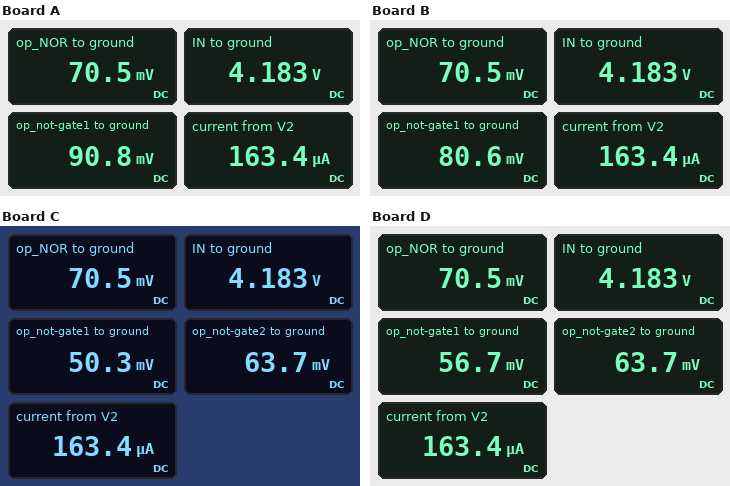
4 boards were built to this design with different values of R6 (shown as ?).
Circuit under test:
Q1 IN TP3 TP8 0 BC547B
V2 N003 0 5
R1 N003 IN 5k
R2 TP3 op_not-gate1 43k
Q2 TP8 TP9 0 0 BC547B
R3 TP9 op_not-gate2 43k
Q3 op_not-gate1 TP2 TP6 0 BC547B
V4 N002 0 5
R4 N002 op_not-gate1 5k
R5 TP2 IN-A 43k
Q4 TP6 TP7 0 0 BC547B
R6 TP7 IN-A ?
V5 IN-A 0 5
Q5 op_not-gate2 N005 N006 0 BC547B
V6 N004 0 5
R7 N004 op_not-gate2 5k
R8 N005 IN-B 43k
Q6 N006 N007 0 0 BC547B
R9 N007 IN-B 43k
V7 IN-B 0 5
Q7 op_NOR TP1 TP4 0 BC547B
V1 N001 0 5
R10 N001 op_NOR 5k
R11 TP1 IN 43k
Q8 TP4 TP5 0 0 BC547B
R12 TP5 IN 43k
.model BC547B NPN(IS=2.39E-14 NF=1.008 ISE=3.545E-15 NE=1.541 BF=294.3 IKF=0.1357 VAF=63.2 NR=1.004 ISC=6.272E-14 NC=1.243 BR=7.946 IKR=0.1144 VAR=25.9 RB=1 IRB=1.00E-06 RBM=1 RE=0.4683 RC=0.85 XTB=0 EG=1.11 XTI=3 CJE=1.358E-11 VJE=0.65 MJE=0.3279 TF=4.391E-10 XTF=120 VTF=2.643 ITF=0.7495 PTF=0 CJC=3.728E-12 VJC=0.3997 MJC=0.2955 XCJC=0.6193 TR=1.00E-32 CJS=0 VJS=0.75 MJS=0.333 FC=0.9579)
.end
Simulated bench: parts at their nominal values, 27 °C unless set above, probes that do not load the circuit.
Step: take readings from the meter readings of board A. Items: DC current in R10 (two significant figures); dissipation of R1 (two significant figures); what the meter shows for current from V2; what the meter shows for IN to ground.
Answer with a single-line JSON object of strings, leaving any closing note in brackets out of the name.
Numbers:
{"DC current in R10": "990 µA", "dissipation of R1": "130 µW", "what the meter shows for current from V2": "163.4 µA", "what the meter shows for IN to ground": "4.183 V"}
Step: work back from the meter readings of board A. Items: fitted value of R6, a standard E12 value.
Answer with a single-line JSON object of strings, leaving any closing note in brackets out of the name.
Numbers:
{"fitted value of R6, a standard E12 value": "150 kΩ"}
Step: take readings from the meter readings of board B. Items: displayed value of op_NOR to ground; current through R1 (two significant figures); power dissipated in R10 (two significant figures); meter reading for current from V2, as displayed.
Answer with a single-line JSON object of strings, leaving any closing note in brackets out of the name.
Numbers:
{"displayed value of op_NOR to ground": "70.5 mV", "current through R1": "160 µA", "power dissipated in R10": "4.9 mW", "meter reading for current from V2, as displayed": "163.4 µA"}
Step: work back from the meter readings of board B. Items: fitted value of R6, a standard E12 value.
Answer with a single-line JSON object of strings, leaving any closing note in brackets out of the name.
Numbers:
{"fitted value of R6, a standard E12 value": "100 kΩ"}
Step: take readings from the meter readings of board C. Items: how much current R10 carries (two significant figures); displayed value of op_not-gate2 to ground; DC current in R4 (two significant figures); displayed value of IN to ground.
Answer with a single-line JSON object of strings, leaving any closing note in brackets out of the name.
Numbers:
{"how much current R10 carries": "990 µA", "displayed value of op_not-gate2 to ground": "63.7 mV", "DC current in R4": "990 µA", "displayed value of IN to ground": "4.183 V"}
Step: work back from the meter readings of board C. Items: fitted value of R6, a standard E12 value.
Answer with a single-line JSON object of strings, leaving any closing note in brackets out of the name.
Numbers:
{"fitted value of R6, a standard E12 value": "15 kΩ"}
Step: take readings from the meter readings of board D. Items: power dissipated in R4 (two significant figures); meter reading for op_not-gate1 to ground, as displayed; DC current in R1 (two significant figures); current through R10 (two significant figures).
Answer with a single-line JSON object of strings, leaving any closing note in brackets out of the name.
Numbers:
{"power dissipated in R4": "4.9 mW", "meter reading for op_not-gate1 to ground, as displayed": "56.7 mV", "DC current in R1": "160 µA", "current through R10": "990 µA"}
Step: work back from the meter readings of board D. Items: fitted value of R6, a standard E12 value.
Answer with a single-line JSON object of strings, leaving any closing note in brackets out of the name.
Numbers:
{"fitted value of R6, a standard E12 value": "27 kΩ"}
